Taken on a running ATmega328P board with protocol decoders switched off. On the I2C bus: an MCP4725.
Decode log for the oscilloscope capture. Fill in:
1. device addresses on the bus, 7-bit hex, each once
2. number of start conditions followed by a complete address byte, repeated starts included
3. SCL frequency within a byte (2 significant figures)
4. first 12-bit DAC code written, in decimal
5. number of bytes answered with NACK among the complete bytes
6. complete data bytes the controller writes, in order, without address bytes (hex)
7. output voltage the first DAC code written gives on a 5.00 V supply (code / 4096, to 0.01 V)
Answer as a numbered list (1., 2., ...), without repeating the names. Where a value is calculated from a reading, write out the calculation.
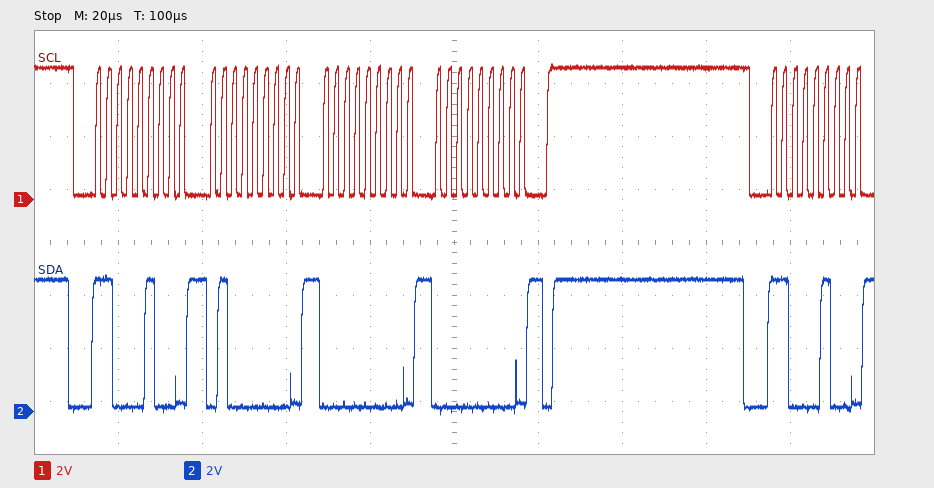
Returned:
1. 0x62
2. 2
3. 400 kHz
4. 0
5. 0
6. 40 00 00
7. 0 / 4096 x 5.00 V = 0.00 V
